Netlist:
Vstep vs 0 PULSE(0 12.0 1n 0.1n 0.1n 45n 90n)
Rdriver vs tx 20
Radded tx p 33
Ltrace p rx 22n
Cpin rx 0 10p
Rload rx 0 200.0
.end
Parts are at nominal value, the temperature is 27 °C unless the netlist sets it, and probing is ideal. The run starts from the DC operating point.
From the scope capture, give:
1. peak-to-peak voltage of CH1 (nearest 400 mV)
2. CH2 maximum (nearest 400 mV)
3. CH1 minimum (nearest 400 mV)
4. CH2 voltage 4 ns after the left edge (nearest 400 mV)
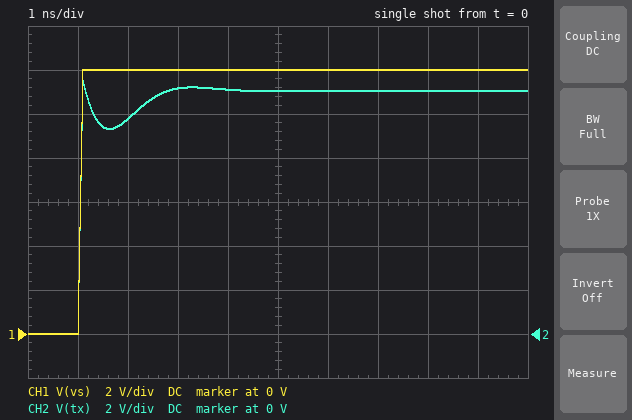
12.0 V
11.6 V
0 V
11.2 V
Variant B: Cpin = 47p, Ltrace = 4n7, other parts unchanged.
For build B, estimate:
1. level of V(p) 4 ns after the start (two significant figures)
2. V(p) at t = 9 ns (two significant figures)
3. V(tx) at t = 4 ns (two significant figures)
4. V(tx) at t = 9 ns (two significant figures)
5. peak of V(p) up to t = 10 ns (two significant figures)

7.3 V
9.3 V
10 V
11 V
9.4 V
